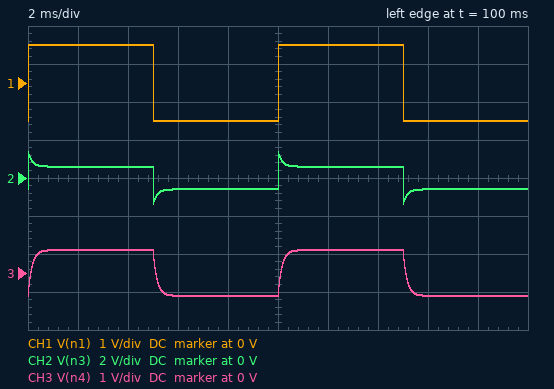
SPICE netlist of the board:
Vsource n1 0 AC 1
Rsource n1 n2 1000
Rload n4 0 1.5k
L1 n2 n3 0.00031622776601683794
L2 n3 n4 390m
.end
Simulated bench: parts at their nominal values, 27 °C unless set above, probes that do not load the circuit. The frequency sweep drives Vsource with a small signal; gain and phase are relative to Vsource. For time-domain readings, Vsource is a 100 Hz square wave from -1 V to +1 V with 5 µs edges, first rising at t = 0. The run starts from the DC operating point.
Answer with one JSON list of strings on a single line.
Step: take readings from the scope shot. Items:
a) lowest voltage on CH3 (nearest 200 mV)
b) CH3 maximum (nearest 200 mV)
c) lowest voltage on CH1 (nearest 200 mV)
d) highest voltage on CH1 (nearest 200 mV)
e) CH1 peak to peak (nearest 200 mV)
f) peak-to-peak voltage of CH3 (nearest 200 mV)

["-600 mV", "600 mV", "-1.0 V", "1.0 V", "2.0 V", "1.2 V"]
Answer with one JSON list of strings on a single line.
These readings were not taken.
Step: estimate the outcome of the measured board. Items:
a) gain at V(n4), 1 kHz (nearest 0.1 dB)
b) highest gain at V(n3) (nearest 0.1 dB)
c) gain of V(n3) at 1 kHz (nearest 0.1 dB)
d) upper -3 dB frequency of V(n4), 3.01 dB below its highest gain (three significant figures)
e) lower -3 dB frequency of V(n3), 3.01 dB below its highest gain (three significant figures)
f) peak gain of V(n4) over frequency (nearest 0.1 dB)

["-7.4 dB", "0 dB", "-1.7 dB", "1.02 kHz", "538 Hz", "-4.4 dB"]
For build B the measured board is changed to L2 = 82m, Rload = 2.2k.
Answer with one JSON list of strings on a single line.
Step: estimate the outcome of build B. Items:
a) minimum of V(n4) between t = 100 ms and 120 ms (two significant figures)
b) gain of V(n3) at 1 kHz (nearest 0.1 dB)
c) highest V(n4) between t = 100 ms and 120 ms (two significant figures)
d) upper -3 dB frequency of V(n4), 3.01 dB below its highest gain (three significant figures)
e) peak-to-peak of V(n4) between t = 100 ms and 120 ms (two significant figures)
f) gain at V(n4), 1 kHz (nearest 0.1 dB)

["-690 mV", "-3.1 dB", "690 mV", "6.19 kHz", "1.4 V", "-3.4 dB"]
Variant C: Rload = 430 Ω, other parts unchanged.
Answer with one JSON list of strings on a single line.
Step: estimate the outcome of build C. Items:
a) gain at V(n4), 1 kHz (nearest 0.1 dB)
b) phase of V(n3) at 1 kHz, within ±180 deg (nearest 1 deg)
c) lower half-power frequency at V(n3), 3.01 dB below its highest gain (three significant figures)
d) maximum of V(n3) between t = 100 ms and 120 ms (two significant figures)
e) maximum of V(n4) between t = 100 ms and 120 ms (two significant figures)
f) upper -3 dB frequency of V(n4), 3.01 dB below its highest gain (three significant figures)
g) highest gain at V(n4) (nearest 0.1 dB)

["-16.4 dB", "20 deg", "528 Hz", "1.7 V", "300 mV", "583 Hz", "-10.4 dB"]
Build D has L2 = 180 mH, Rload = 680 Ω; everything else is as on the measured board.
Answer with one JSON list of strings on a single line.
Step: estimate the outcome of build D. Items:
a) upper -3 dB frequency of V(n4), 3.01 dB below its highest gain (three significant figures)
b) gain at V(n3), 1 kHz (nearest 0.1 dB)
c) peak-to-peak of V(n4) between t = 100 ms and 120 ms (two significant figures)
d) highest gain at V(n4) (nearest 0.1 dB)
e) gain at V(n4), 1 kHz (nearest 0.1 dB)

["1.48 kHz", "-3.7 dB", "810 mV", "-7.9 dB", "-9.5 dB"]
